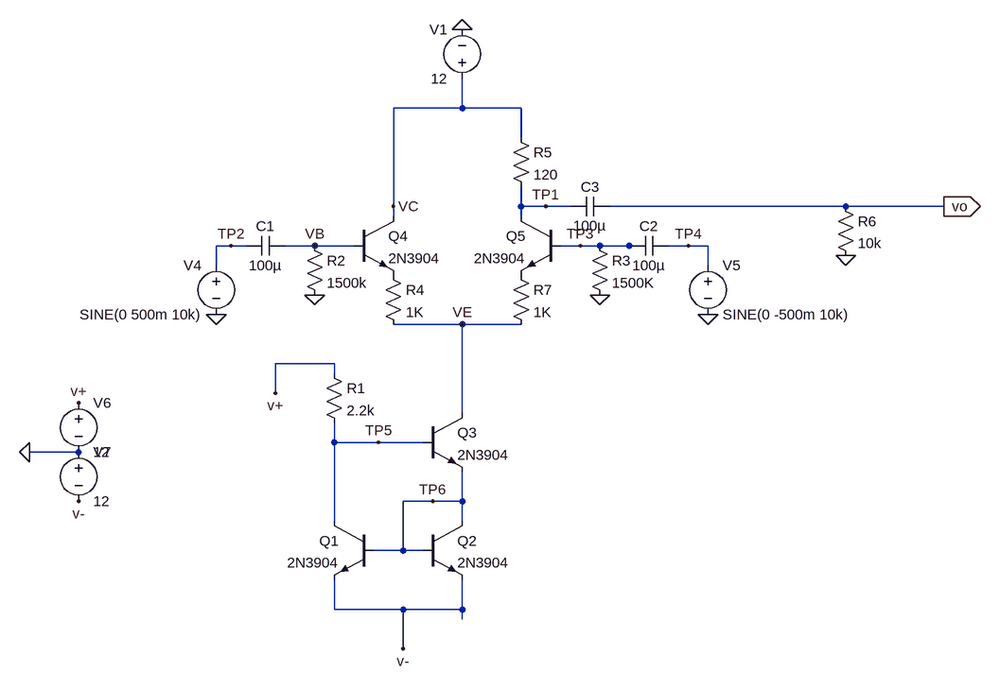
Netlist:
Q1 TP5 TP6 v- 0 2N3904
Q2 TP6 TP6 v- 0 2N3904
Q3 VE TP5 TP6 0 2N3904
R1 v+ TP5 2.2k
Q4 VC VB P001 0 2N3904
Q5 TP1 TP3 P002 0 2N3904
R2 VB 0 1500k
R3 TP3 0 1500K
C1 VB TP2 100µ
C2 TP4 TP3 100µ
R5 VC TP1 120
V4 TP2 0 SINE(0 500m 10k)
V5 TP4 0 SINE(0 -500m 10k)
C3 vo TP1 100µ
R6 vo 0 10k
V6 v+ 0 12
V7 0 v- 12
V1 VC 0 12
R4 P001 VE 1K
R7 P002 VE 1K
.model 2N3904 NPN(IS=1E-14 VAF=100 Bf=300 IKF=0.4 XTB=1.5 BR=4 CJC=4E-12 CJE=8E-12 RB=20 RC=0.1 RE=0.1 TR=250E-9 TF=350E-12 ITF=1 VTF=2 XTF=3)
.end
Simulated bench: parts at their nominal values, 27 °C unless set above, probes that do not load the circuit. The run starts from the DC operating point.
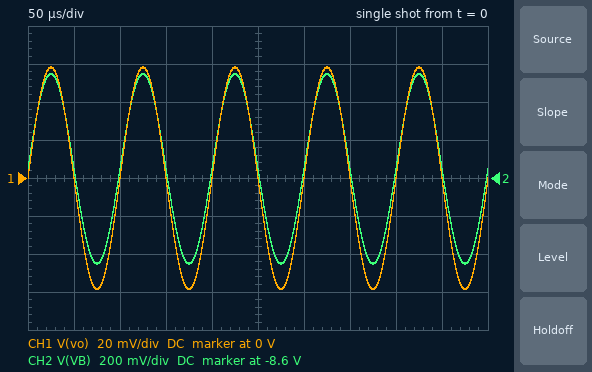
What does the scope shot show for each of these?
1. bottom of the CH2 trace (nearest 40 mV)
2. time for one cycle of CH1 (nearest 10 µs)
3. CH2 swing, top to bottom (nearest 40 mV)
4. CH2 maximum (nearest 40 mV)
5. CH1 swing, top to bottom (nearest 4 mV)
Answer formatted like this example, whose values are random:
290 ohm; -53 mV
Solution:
-9.04 V; 100 µs; 1.00 V; -8.04 V; 116 mV
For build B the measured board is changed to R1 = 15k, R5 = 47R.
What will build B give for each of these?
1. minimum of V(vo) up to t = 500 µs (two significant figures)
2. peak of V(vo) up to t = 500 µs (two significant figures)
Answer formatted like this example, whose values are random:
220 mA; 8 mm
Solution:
-22 mV; 22 mV
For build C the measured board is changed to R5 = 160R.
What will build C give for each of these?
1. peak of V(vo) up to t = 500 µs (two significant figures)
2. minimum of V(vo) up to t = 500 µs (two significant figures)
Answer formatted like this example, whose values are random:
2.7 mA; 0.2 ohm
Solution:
77 mV; -78 mV
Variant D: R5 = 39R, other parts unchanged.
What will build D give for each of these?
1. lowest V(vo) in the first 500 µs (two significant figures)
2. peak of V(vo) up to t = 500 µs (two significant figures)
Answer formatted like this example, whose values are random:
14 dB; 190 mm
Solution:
-19 mV; 19 mV
